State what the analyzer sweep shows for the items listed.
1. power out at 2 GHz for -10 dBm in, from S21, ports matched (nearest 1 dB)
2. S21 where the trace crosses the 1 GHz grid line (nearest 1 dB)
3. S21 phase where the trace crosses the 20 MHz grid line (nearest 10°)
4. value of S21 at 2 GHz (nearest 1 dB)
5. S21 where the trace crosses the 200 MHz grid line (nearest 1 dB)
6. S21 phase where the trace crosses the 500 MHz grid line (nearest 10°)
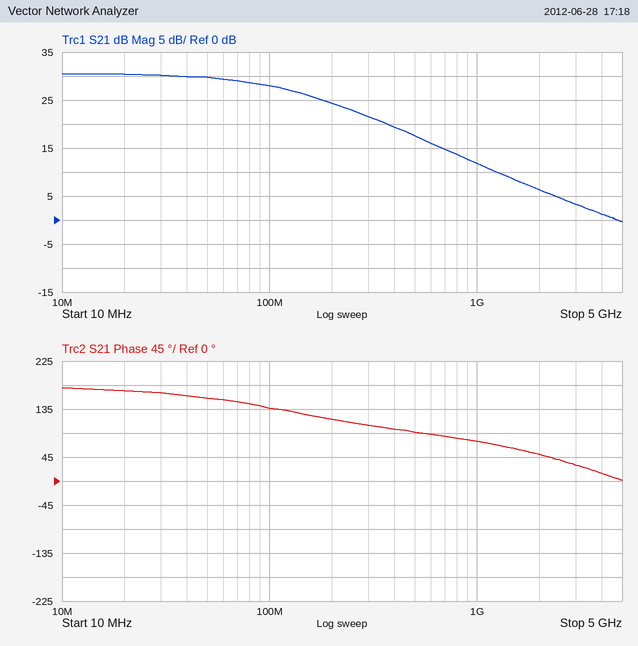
-4 dBm
12 dB
170°
6 dB
24 dB
90°
